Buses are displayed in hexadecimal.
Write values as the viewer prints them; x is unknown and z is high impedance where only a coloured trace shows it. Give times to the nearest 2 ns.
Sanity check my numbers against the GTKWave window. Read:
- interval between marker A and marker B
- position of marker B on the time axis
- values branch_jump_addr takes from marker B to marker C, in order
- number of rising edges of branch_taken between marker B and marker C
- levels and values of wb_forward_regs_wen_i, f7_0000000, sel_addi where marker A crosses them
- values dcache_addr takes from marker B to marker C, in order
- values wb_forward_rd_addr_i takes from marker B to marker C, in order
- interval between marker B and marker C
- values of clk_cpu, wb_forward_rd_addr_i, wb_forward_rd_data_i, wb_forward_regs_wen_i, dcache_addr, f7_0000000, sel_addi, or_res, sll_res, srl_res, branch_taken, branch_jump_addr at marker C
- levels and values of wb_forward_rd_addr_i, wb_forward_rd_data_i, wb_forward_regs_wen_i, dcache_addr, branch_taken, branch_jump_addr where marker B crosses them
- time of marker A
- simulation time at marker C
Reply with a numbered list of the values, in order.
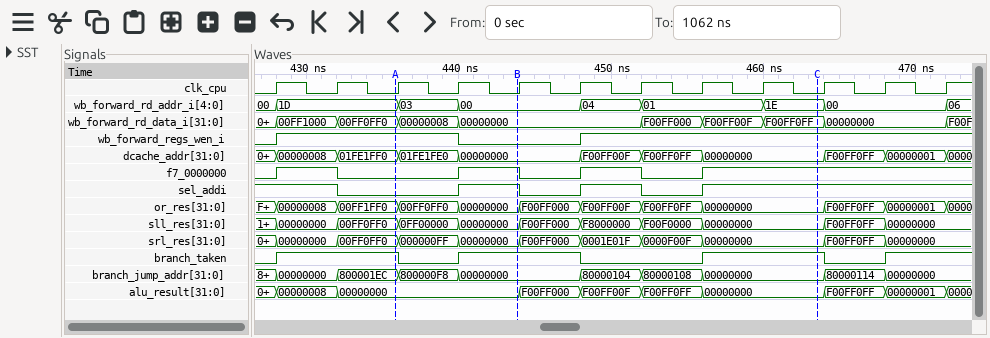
1. 8 ns
2. 444 ns
3. 00000000, 80000104, 80000108, 00000000
4. 1
5. wb_forward_regs_wen_i=1, f7_0000000=0, sel_addi=0
6. 00000000, F00FF00F, F00FF0FF, 00000000
7. 00, 04, 01, 1E
8. 20 ns
9. clk_cpu=0, wb_forward_rd_addr_i=1E, wb_forward_rd_data_i=F00FF0FF, wb_forward_regs_wen_i=1, dcache_addr=00000000, f7_0000000=1, sel_addi=1, or_res=00000000, sll_res=00000000, srl_res=00000000, branch_taken=1, branch_jump_addr=00000000
10. wb_forward_rd_addr_i=00, wb_forward_rd_data_i=00000000, wb_forward_regs_wen_i=0, dcache_addr=00000000, branch_taken=1, branch_jump_addr=00000000
11. 436 ns
12. 464 ns
